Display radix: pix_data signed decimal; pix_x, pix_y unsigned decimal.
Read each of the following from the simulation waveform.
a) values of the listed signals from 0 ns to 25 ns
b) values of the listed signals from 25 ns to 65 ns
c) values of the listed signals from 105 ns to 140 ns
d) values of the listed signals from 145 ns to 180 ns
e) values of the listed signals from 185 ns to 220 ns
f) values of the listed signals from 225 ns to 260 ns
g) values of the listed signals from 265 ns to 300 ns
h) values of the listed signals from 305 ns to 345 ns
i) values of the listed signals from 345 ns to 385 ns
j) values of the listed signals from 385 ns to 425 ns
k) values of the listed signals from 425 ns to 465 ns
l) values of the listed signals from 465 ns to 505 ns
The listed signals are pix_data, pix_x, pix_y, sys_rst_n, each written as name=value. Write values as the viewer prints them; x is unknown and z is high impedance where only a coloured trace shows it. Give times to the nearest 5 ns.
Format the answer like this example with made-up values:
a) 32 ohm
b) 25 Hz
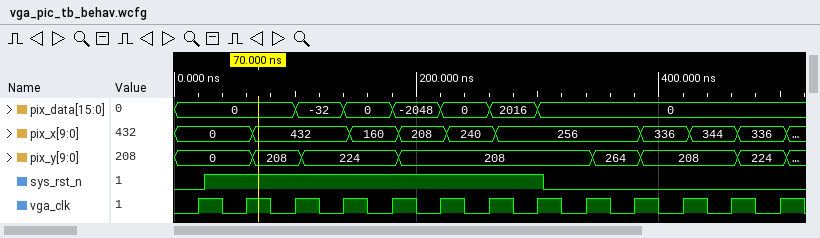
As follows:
a) pix_data=0, pix_x=0, pix_y=0, sys_rst_n=0
b) pix_data=0, pix_x=0, pix_y=0, sys_rst_n=1
c) pix_data=-32, pix_x=432, pix_y=224, sys_rst_n=1
d) pix_data=0, pix_x=160, pix_y=224, sys_rst_n=1
e) pix_data=-2048, pix_x=208, pix_y=208, sys_rst_n=1
f) pix_data=0, pix_x=240, pix_y=208, sys_rst_n=1
g) pix_data=2016, pix_x=256, pix_y=208, sys_rst_n=1
h) pix_data=0, pix_x=256, pix_y=208, sys_rst_n=0
i) pix_data=0, pix_x=256, pix_y=264, sys_rst_n=0
j) pix_data=0, pix_x=336, pix_y=208, sys_rst_n=0
k) pix_data=0, pix_x=344, pix_y=208, sys_rst_n=0
l) pix_data=0, pix_x=336, pix_y=224, sys_rst_n=0
